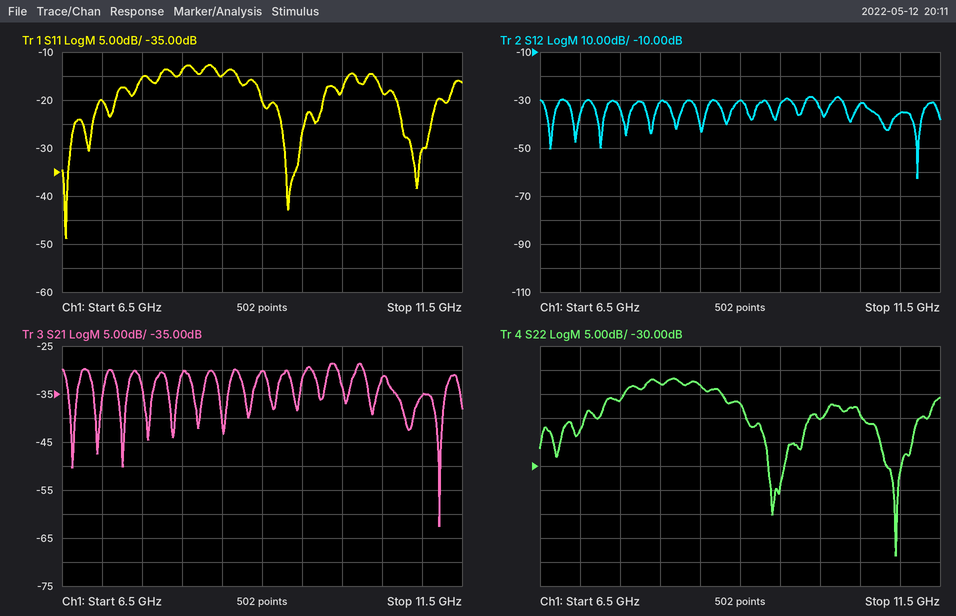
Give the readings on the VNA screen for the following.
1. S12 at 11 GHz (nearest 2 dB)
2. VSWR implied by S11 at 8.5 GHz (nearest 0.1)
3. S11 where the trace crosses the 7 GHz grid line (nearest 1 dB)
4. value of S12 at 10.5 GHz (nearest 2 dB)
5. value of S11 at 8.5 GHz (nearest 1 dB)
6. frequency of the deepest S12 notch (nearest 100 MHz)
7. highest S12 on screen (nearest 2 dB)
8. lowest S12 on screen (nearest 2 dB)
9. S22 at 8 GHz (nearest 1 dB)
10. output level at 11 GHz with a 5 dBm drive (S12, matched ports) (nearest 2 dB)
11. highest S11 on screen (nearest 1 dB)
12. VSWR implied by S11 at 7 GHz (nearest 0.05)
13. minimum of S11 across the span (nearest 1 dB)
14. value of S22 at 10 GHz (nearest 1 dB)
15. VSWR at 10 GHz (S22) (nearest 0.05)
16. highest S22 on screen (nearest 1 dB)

-36 dB
1.4
-20 dB
-32 dB
-15 dB
11.2 GHz
-28 dB
-62 dB
-13 dB
-30 dBm
-13 dB
1.20
-49 dB
-20 dB
1.20
-12 dB
